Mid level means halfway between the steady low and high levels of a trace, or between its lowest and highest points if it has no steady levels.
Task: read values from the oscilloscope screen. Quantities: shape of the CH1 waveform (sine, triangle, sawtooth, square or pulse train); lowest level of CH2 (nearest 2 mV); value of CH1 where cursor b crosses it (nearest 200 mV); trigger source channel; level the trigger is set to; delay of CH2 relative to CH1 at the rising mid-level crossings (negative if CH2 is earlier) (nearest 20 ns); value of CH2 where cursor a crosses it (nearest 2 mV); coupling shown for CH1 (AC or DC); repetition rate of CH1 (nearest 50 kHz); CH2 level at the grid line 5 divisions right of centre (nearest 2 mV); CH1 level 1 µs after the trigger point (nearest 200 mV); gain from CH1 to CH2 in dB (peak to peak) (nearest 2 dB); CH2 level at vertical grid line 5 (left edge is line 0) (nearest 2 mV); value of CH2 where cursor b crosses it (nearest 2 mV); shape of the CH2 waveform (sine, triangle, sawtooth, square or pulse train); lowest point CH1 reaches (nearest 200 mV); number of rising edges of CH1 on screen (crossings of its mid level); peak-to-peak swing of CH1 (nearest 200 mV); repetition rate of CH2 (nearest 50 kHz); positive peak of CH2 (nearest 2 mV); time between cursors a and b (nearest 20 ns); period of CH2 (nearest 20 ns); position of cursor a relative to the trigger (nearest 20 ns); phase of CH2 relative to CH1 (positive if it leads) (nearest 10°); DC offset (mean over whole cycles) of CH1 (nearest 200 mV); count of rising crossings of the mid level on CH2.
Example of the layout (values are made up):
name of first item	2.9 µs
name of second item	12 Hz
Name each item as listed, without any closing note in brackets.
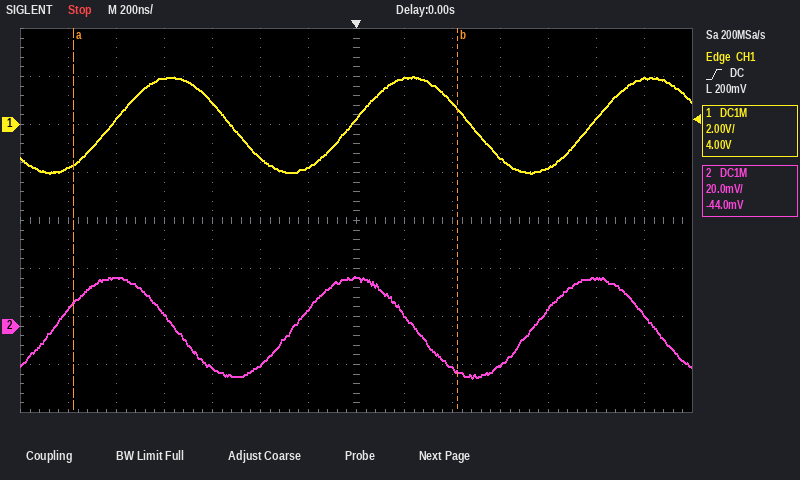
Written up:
shape of the CH1 waveform	sine
lowest level of CH2	-22 mV
value of CH1 where cursor b crosses it	600 mV
trigger source channel	CH1
level the trigger is set to	200 mV
delay of CH2 relative to CH1 at the rising mid-level crossings (negative if CH2 is earlier)	-240 ns
value of CH2 where cursor a crosses it	10 mV
coupling shown for CH1	DC
repetition rate of CH1	1.00 MHz
CH2 level at the grid line 5 divisions right of centre	20 mV
CH1 level 1 µs after the trigger point	200 mV
gain from CH1 to CH2 in dB (peak to peak)	-40 dB
CH2 level at vertical grid line 5 (left edge is line 0)	-16 mV
value of CH2 where cursor b crosses it	-18 mV
shape of the CH2 waveform	sine
lowest point CH1 reaches	-2.0 V
number of rising edges of CH1 on screen	3
peak-to-peak swing of CH1	4.0 V
repetition rate of CH2	1.00 MHz
positive peak of CH2	20 mV
time between cursors a and b	1.60 µs
period of CH2	1.00 µs
position of cursor a relative to the trigger	-1.18 µs
phase of CH2 relative to CH1 (positive if it leads)	+90°
DC offset (mean over whole cycles) of CH1	0.0 V
count of rising crossings of the mid level on CH2	3
